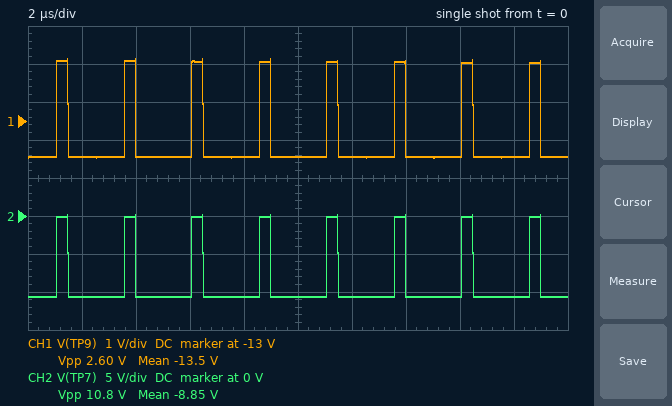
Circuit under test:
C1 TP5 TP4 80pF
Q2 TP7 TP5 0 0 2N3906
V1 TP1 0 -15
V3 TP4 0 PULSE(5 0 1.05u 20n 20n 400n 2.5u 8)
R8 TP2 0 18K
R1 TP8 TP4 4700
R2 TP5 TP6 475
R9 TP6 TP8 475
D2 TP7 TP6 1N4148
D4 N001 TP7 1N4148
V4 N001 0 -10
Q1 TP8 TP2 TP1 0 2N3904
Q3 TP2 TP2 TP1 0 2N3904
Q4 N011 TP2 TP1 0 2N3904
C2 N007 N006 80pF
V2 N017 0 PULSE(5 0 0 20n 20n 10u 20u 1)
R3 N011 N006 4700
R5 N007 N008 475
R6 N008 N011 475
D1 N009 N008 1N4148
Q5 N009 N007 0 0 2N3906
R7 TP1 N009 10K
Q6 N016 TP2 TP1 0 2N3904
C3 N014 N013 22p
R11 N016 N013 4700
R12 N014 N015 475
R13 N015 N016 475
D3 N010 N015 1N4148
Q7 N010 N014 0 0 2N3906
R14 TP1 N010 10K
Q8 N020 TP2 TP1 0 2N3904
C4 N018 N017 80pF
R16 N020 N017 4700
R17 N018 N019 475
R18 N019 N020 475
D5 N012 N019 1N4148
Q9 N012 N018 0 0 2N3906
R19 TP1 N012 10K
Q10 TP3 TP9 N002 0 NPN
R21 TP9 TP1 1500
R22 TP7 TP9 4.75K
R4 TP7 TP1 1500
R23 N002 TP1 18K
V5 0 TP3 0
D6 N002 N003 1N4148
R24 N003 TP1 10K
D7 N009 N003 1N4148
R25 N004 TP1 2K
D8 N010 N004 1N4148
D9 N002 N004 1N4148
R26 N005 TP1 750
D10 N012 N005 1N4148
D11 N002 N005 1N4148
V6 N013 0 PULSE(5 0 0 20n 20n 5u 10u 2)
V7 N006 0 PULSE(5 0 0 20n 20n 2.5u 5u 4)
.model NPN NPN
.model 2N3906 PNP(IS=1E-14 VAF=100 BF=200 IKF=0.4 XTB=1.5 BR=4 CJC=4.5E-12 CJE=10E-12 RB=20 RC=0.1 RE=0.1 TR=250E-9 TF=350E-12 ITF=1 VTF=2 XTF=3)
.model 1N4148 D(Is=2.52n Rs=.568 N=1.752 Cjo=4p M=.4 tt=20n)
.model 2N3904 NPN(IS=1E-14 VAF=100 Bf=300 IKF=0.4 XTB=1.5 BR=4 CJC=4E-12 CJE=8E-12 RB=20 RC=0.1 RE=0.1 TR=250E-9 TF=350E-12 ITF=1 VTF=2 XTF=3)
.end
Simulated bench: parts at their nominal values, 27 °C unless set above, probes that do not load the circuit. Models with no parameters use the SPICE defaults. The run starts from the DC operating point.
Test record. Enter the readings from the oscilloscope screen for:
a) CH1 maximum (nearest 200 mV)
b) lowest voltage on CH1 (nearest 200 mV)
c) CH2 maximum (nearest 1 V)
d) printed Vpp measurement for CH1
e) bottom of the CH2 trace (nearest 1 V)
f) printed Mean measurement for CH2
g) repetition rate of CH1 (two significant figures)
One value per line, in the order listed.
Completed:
-11.4 V
-14.0 V
0 V
2.60 V
-11 V
-8.85 V
400 kHz
